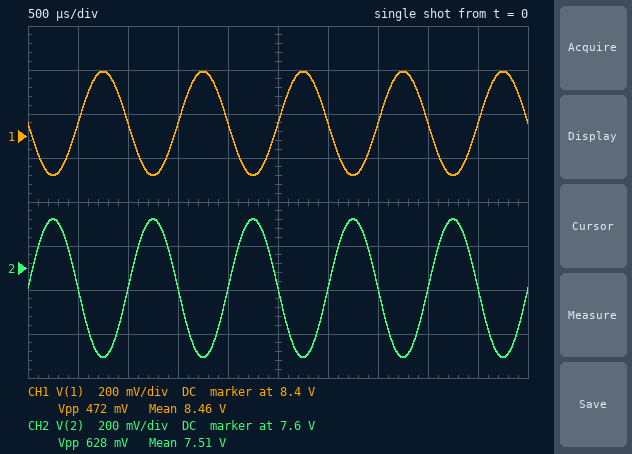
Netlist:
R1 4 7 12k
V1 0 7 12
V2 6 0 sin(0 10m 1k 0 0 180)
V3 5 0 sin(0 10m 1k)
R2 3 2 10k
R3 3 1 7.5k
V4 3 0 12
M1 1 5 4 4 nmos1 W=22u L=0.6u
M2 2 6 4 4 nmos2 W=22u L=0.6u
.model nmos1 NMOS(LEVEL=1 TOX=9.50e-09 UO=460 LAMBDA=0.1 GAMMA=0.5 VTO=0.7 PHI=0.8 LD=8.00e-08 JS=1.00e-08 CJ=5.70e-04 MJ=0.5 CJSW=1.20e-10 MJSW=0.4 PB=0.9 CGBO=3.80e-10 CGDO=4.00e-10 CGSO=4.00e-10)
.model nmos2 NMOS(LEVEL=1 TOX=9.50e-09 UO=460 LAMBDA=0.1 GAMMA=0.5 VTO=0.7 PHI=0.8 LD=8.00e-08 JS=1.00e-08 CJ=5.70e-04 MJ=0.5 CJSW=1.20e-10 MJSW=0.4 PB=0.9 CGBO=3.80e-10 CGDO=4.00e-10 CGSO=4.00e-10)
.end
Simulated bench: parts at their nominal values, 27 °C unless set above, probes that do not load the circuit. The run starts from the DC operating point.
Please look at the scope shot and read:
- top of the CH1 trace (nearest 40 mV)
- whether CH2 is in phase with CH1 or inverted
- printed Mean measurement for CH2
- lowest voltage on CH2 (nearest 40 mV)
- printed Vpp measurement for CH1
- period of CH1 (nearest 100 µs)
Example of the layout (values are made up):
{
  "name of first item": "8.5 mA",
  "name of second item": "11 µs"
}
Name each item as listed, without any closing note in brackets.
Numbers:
{
  "top of the CH1 trace": "8.68 V",
  "whether CH2 is in phase with CH1 or inverted": "inverted",
  "printed Mean measurement for CH2": "7.51 V",
  "lowest voltage on CH2": "7.20 V",
  "printed Vpp measurement for CH1": "472 mV",
  "period of CH1": "1.0 ms"
}
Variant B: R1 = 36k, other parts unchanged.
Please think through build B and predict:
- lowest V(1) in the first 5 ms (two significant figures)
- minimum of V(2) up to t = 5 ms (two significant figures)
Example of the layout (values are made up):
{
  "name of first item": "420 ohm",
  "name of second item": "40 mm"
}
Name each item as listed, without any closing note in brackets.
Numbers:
{
  "lowest V(1) in the first 5 ms": "11 V",
  "minimum of V(2) up to t = 5 ms": "10 V"
}
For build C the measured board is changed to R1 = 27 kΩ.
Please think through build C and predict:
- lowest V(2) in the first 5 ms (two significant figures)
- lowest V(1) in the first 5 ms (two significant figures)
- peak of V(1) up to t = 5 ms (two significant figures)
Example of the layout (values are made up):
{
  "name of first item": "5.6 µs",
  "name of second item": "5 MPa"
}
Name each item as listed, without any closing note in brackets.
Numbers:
{
  "lowest V(2) in the first 5 ms": "9.7 V",
  "lowest V(1) in the first 5 ms": "10 V",
  "peak of V(1) up to t = 5 ms": "11 V"
}
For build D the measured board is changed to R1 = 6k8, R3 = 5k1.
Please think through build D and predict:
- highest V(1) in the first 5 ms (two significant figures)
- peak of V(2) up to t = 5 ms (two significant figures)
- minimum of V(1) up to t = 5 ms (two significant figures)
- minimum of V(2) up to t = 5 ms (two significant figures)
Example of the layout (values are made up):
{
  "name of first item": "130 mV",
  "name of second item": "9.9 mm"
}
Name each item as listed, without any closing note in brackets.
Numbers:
{
  "highest V(1) in the first 5 ms": "7.7 V",
  "peak of V(2) up to t = 5 ms": "5.0 V",
  "minimum of V(1) up to t = 5 ms": "7.4 V",
  "minimum of V(2) up to t = 5 ms": "4.3 V"
}
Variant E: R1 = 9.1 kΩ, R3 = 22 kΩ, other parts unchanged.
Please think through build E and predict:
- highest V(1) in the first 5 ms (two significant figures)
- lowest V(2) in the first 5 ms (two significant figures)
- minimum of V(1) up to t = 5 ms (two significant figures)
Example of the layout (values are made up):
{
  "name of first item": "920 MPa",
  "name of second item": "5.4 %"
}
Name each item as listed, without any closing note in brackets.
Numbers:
{
  "highest V(1) in the first 5 ms": "1.2 V",
  "lowest V(2) in the first 5 ms": "4.8 V",
  "minimum of V(1) up to t = 5 ms": "310 mV"
}
